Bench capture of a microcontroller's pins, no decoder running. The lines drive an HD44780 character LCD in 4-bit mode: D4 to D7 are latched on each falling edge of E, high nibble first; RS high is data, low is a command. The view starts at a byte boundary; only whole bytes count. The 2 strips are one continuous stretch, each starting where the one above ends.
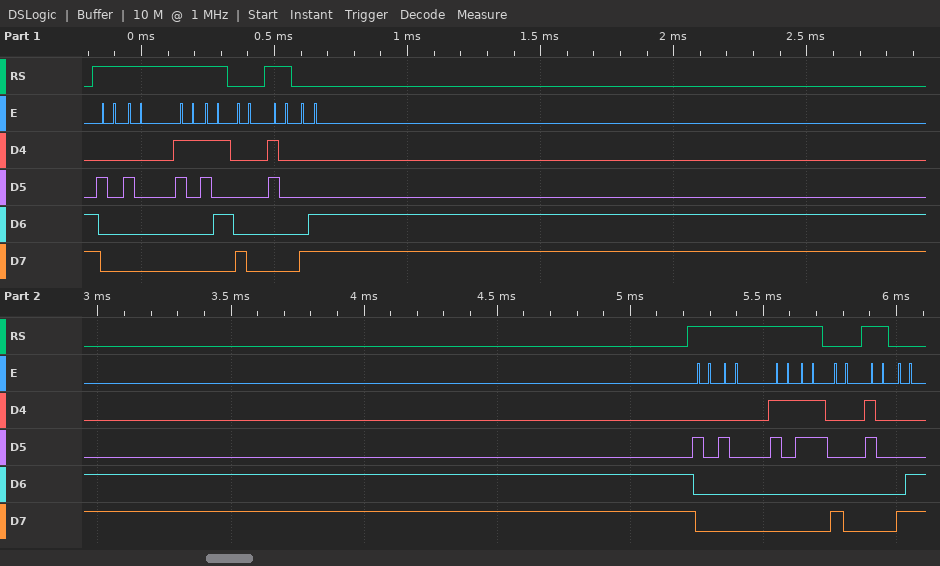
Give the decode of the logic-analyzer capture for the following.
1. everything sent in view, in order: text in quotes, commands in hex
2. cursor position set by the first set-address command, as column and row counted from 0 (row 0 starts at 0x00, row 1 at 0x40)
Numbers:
"  15" 0x80 "0" 0x8C "  13" 0x80 "0" 0x8C
column 0, row 0
